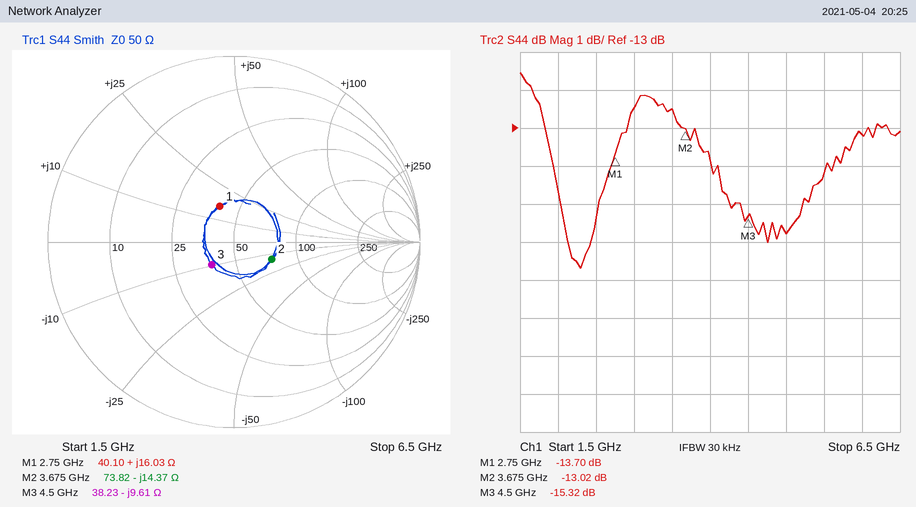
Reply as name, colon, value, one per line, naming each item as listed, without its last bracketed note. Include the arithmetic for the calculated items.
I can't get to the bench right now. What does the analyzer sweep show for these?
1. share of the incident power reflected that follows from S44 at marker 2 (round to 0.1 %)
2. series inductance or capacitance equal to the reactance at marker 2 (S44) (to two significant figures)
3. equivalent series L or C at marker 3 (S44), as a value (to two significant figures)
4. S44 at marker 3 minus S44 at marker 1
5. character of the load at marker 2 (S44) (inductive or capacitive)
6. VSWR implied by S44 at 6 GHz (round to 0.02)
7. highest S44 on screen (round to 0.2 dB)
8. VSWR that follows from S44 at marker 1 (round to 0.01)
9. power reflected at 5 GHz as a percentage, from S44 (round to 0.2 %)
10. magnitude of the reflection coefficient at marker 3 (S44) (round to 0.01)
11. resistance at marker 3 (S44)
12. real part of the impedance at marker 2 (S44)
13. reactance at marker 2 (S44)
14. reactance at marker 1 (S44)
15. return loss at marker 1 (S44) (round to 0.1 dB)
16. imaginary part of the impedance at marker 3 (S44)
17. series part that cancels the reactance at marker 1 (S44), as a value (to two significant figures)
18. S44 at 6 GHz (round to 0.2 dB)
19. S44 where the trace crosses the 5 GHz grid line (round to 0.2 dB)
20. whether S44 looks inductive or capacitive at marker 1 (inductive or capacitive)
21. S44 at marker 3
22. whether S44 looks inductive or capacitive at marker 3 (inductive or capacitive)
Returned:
share of the incident power reflected that follows from S44 at marker 2: 10^(-13.02/10) ≈ 5.0 %
series inductance or capacitance equal to the reactance at marker 2 (S44): C = 1/(2π × 3.675 GHz × 14.37 Ω) ≈ 3.0 pF
equivalent series L or C at marker 3 (S44), as a value: C = 1/(2π × 4.5 GHz × 9.61 Ω) ≈ 3.7 pF
S44 at marker 3 minus S44 at marker 1: -15.32 − (-13.7) = -1.62 dB
character of the load at marker 2 (S44): capacitive
VSWR implied by S44 at 6 GHz: |Γ| = 10^(-13.2/20) = 0.2188; VSWR = (1 + 0.2188)/(1 − 0.2188) ≈ 1.56
highest S44 on screen: -11.6 dB
VSWR that follows from S44 at marker 1: (1 + 0.2065)/(1 − 0.2065) ≈ 1.52
power reflected at 5 GHz as a percentage, from S44: 10^(-15.8/10) ≈ 2.6 %
magnitude of the reflection coefficient at marker 3 (S44): 0.17
resistance at marker 3: 38.23 Ω
real part of the impedance at marker 2: 73.82 Ω
reactance at marker 2: -14.37 Ω
reactance at marker 1: +16.03 Ω
return loss at marker 1 (S44): 13.7 dB
imaginary part of the impedance at marker 3: -9.61 Ω
series part that cancels the reactance at marker 1 (S44), as a value: C = 1/(2π × 2.75 GHz × 16.03 Ω) ≈ 3.6 pF
S44 at 6 GHz: -13.2 dB
S44 where the trace crosses the 5 GHz grid line: -15.8 dB
whether S44 looks inductive or capacitive at marker 1: inductive
S44 at marker 3: -15.32 dB
whether S44 looks inductive or capacitive at marker 3: capacitive
